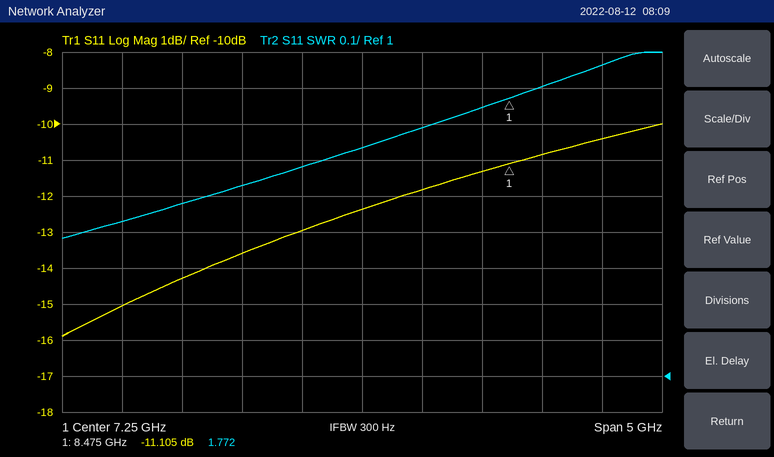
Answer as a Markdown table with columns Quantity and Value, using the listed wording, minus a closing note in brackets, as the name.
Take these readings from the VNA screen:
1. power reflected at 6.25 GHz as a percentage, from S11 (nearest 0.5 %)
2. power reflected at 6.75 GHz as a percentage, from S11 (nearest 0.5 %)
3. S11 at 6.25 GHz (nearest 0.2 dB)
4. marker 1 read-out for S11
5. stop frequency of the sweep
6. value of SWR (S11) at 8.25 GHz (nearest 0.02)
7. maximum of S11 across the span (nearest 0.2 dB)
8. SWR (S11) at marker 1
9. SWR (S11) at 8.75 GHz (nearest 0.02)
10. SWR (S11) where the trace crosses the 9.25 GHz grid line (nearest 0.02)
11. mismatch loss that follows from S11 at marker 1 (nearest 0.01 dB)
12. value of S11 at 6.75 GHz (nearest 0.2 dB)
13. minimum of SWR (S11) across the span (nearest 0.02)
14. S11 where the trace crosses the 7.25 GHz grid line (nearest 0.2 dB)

| Quantity | Value |
|---|---|
| power reflected at 6.25 GHz as a percentage, from S11 | 4.5 % |
| power reflected at 6.75 GHz as a percentage, from S11 | 5.0 % |
| S11 at 6.25 GHz | -13.6 dB |
| marker 1 read-out for S11 | -11.105 dB |
| stop frequency of the sweep | 9.75 GHz |
| value of SWR (S11) at 8.25 GHz | 1.74 |
| maximum of S11 across the span | -10.0 dB |
| SWR (S11) at marker 1 | 1.772 |
| SWR (S11) at 8.75 GHz | 1.80 |
| SWR (S11) where the trace crosses the 9.25 GHz grid line | 1.86 |
| mismatch loss that follows from S11 at marker 1 | 0.35 dB |
| value of S11 at 6.75 GHz | -13.0 dB |
| minimum of SWR (S11) across the span | 1.38 |
| S11 where the trace crosses the 7.25 GHz grid line | -12.4 dB |
